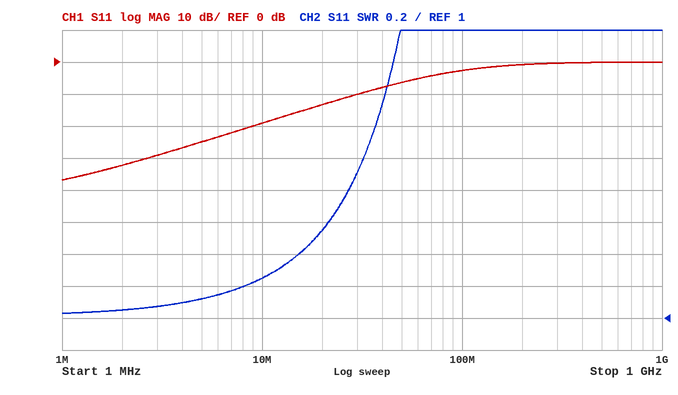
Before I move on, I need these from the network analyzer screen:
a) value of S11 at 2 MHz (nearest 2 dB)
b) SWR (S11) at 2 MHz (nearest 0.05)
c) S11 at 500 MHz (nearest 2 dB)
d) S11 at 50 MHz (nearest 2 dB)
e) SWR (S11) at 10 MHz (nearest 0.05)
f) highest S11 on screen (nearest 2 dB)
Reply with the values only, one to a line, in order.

-32 dB
1.05
0 dB
-6 dB
1.25
0 dB
